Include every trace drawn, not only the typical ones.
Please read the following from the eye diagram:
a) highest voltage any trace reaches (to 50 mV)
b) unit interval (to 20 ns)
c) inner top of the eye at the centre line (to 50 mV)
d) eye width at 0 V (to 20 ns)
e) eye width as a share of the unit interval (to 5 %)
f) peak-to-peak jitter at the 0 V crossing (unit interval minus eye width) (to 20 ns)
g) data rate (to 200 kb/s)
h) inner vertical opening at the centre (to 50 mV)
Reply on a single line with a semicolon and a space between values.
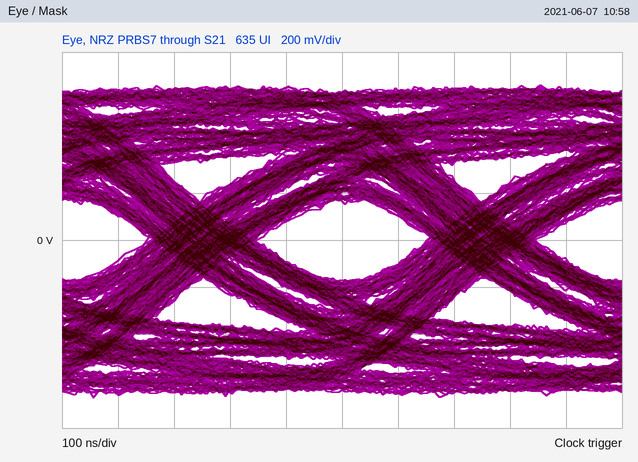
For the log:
650 mV; 500 ns; 150 mV; 300 ns; 60 %; 200 ns; 2.0 Mb/s; 350 mV
